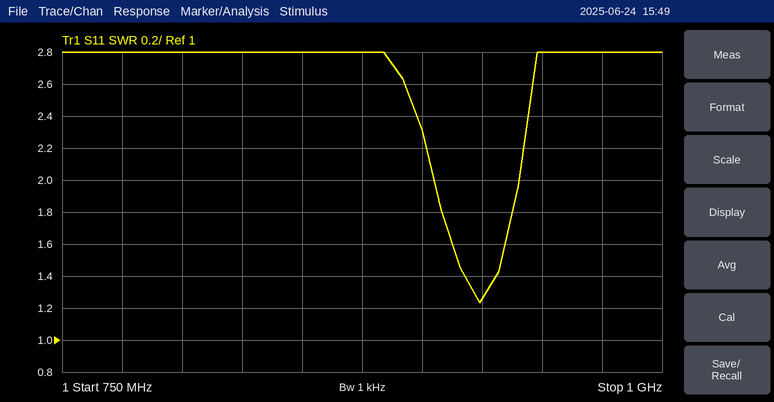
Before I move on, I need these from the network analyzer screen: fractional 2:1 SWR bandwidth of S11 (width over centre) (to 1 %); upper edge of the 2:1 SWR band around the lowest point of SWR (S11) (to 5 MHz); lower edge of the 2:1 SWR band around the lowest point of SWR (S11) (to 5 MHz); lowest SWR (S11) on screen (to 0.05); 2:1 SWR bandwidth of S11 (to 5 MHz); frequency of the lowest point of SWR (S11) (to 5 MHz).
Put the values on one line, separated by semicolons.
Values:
4 %; 940 MHz; 905 MHz; 1.25; 35 MHz; 925 MHz
